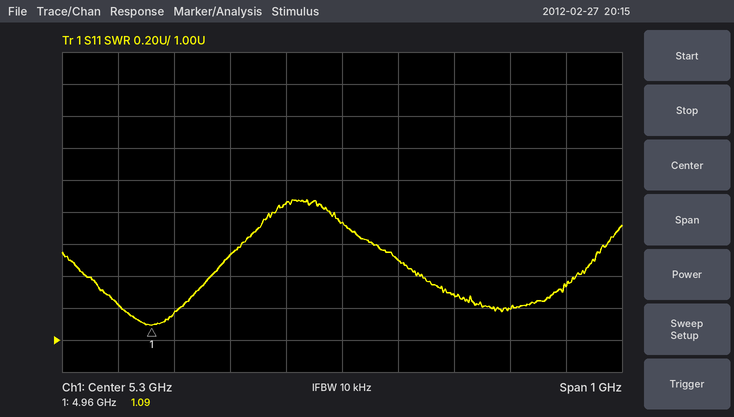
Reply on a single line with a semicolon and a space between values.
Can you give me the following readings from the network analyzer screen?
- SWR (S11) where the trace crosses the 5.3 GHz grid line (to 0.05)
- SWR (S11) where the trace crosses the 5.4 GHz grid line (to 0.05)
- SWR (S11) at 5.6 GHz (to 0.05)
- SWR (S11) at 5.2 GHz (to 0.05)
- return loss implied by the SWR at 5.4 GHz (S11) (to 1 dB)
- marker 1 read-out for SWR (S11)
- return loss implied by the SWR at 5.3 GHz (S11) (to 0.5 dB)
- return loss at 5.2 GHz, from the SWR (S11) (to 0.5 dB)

1.75; 1.50; 1.20; 1.85; 14 dB; 1.09; 11.5 dB; 10.5 dB
